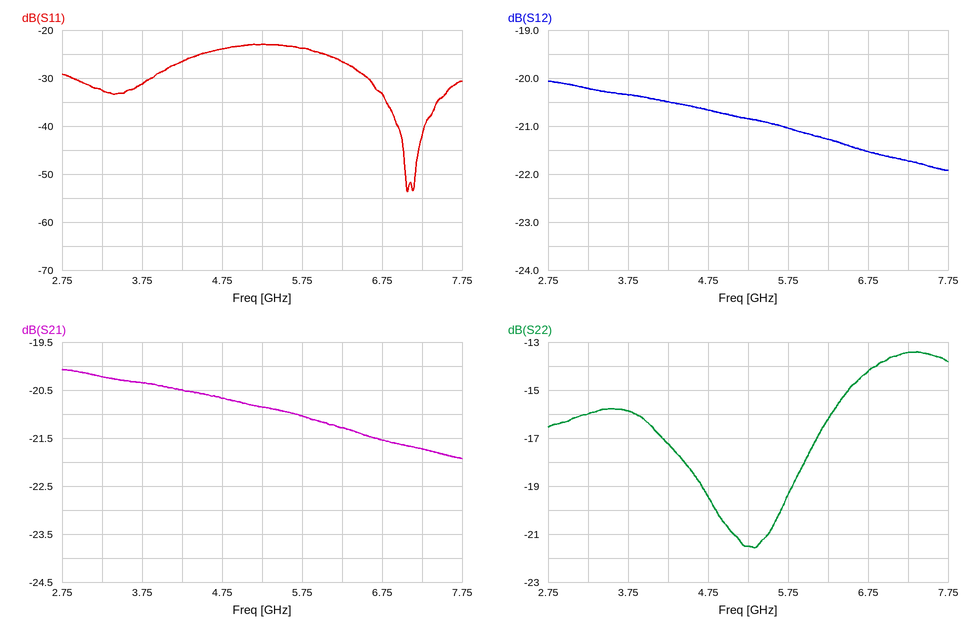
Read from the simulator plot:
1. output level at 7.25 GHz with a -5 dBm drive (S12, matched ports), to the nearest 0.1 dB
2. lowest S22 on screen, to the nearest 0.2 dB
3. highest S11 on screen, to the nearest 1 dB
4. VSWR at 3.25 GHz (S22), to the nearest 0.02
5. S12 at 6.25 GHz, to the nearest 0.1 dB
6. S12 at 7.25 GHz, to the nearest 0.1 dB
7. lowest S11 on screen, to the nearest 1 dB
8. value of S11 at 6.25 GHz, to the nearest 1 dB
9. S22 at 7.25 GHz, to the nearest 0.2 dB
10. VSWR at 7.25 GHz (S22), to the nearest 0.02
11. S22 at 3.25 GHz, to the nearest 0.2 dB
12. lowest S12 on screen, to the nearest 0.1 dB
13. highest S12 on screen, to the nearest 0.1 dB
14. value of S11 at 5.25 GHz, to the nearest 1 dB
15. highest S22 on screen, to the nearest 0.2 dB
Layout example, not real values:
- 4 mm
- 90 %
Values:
- -26.7 dBm
- -21.6 dB
- -23 dB
- 1.38
- -21.3 dB
- -21.7 dB
- -54 dB
- -27 dB
- -13.4 dB
- 1.54
- -16.0 dB
- -21.9 dB
- -20.1 dB
- -23 dB
- -13.4 dB
